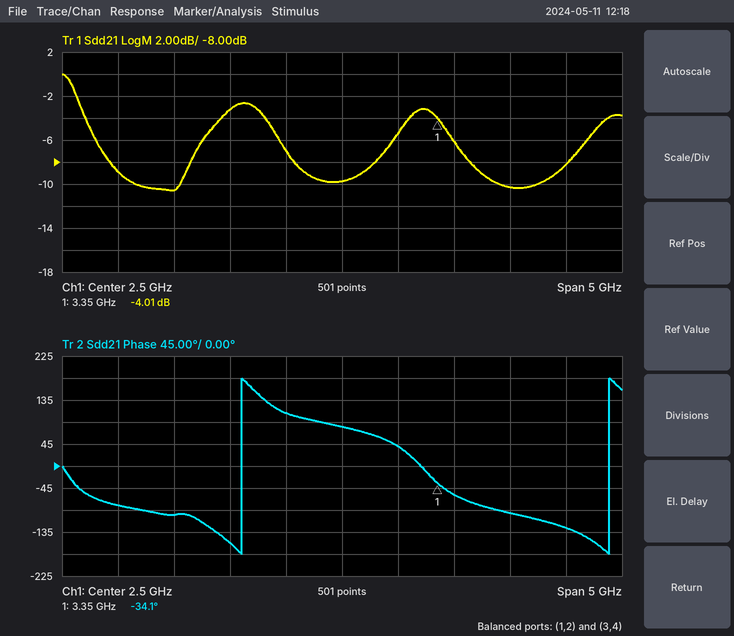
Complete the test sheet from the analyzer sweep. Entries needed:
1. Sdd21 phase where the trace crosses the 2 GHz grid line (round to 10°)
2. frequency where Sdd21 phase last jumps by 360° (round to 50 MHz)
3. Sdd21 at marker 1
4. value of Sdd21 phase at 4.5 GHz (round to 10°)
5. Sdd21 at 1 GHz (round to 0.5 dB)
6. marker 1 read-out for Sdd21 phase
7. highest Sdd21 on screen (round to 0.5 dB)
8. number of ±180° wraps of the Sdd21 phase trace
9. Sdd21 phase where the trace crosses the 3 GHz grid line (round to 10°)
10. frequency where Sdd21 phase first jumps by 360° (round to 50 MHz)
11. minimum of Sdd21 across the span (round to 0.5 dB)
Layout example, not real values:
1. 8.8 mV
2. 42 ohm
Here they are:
1. 110°
2. 4.90 GHz
3. -4.01 dB
4. -130°
5. -10.5 dB
6. -34.1°
7. 0.0 dB
8. 2
9. 40°
10. 1.60 GHz
11. -10.5 dB
